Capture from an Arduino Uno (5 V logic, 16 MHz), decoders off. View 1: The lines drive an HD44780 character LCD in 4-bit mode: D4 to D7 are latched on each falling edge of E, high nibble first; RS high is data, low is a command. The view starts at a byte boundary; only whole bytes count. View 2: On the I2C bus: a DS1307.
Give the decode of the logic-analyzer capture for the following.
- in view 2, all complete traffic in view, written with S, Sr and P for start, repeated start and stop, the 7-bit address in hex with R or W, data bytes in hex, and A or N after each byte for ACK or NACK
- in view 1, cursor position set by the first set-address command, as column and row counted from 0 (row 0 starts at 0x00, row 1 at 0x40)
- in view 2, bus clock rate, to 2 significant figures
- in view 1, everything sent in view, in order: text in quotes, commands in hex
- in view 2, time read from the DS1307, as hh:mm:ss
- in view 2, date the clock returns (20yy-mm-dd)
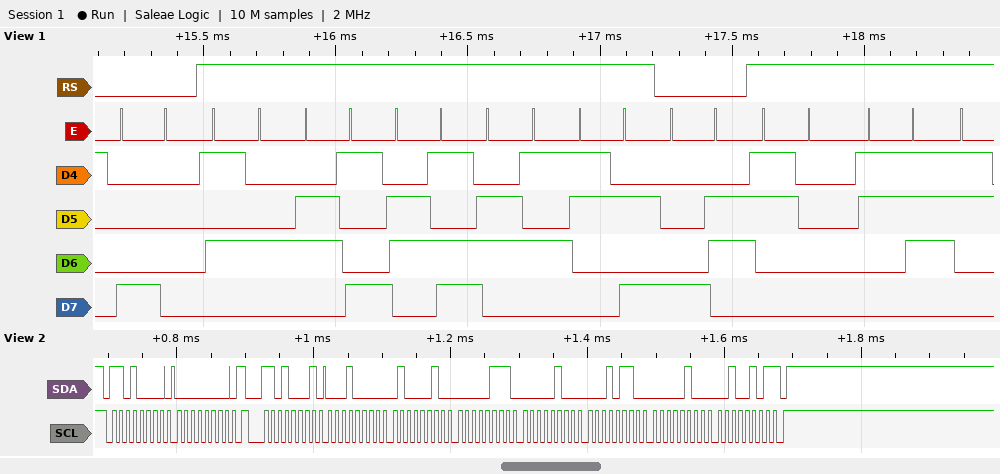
S 68W A 00 A Sr 68R A 10 A 42 A 07 A 04 A 16 A 04 A 25 N P
column 0, row 0
100 kHz
0x80 "Time:" 0x86 "07"
07:42:10
2025-04-16
